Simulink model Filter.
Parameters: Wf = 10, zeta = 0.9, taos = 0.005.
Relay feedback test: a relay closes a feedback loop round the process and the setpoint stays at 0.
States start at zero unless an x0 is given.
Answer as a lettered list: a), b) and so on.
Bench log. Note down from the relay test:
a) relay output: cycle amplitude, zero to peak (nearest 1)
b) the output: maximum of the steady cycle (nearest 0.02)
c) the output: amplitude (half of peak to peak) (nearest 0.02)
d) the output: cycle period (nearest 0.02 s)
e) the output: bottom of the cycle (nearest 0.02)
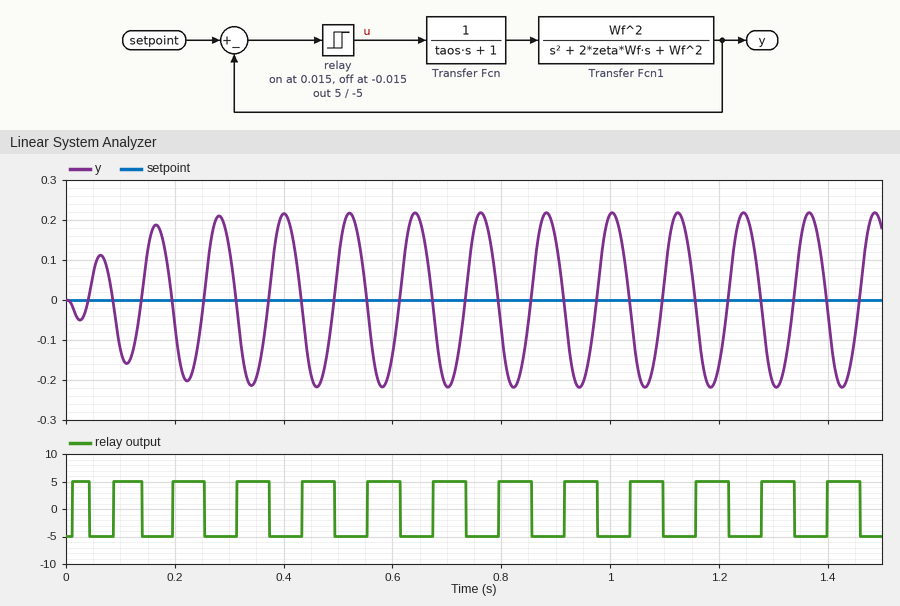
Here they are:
a) 5
b) 0.22
c) 0.22
d) 0.12 s
e) -0.22
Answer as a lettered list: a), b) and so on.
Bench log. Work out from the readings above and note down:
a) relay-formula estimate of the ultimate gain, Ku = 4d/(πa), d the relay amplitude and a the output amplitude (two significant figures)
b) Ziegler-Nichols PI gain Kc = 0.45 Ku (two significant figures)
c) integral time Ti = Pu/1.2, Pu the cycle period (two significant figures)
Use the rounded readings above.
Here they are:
a) 29
b) 13
c) 0.10 s
